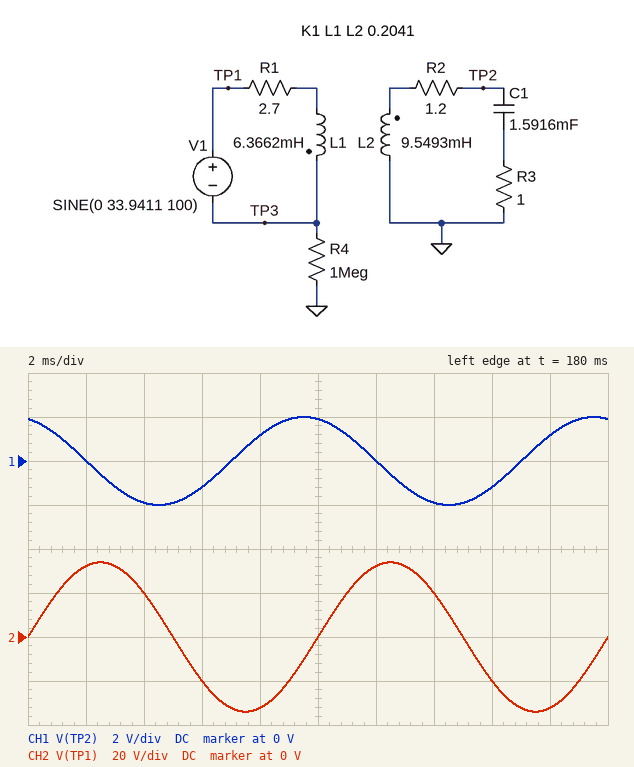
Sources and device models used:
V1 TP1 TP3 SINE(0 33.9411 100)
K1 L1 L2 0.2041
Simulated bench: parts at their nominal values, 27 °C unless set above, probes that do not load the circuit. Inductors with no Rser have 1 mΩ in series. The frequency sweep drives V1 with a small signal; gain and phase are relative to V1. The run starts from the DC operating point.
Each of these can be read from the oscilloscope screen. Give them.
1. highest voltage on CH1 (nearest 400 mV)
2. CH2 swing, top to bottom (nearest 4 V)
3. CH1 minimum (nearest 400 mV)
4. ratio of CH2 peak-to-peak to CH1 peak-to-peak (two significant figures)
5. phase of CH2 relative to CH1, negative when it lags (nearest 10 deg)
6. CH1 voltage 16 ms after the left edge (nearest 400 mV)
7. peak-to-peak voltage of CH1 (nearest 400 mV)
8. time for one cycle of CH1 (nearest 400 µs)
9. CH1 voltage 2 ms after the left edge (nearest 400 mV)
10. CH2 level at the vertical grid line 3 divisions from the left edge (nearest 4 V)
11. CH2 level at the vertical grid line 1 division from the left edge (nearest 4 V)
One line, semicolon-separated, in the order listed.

2.0 V; 68 V; -2.0 V; 17; -110 deg; -1.2 V; 4.0 V; 10.0 ms; 0 V; -20 V; 32 V
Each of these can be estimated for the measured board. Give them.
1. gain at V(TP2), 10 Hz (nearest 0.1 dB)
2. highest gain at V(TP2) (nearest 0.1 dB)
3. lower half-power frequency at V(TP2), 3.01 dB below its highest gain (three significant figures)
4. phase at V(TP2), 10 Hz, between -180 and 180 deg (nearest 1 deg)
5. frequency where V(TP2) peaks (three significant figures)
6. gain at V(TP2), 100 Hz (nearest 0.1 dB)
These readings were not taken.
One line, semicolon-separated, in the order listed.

-28.7 dB; -18.0 dB; 24.9 Hz; -110 deg; 45.0 Hz; -24.6 dB
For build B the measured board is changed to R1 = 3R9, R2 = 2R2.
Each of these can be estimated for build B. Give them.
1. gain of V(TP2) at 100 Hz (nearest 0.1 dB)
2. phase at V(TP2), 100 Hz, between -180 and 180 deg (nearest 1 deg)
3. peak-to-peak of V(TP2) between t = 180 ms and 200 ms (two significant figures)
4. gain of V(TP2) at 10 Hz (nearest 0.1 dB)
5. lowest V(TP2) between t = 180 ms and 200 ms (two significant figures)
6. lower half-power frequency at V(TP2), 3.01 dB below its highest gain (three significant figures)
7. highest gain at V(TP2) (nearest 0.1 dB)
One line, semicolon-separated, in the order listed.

-26.9 dB; 127 deg; 3.1 V; -32.0 dB; -1.5 V; 21.5 Hz; -23.0 dB
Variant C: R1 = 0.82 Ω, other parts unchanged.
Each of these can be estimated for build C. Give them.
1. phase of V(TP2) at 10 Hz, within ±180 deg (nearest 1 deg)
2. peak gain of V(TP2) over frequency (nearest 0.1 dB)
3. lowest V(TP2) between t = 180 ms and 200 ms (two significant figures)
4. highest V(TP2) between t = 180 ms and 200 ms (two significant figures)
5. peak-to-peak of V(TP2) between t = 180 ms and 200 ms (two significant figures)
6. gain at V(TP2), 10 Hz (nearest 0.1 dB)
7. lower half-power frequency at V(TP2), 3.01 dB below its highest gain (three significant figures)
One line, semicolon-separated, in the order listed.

-133 deg; -15.1 dB; -2.2 V; 2.2 V; 4.4 V; -20.0 dB; 14.2 Hz
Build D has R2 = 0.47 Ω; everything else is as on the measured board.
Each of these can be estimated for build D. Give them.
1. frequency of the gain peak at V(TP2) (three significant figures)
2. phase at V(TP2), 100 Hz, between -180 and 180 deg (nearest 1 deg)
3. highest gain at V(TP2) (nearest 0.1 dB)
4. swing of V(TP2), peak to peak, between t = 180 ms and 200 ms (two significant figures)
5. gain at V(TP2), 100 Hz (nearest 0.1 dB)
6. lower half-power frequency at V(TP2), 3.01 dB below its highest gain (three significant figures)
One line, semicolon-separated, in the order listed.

47.8 Hz; 97 deg; -14.7 dB; 4.5 V; -23.6 dB; 31.5 Hz
